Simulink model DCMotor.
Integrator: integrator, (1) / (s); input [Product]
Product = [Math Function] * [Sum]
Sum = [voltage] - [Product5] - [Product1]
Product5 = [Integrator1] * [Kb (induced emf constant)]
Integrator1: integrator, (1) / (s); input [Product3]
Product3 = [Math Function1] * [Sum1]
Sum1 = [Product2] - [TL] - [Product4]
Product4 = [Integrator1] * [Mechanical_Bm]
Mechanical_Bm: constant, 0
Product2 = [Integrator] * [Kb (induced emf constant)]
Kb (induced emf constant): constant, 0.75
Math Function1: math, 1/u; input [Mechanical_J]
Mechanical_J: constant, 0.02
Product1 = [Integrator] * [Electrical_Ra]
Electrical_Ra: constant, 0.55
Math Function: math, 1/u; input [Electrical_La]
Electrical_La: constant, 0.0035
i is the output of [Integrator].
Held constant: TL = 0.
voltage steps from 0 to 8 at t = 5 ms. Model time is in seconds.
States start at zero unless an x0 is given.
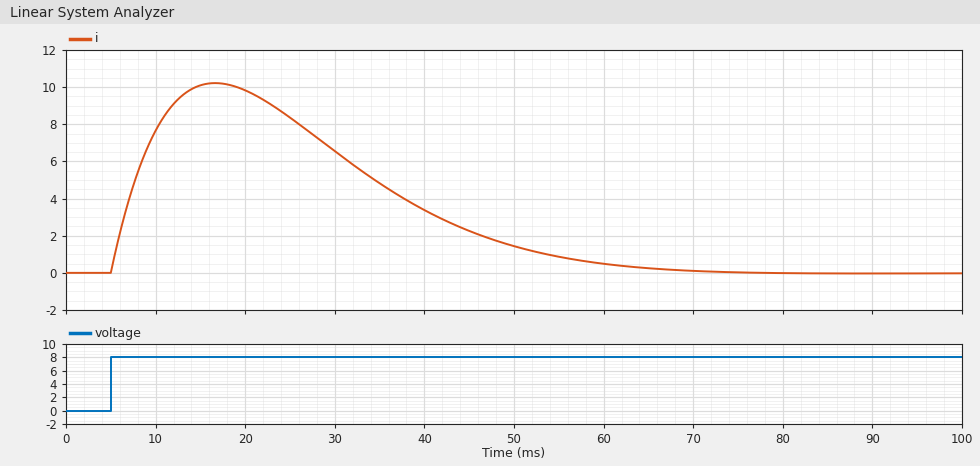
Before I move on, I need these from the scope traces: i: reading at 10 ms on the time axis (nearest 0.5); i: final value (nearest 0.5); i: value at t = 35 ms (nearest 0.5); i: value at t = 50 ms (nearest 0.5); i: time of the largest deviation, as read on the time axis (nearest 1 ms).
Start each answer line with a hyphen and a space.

- 7.5
- 0.0
- 5.0
- 1.5
- 17 ms
